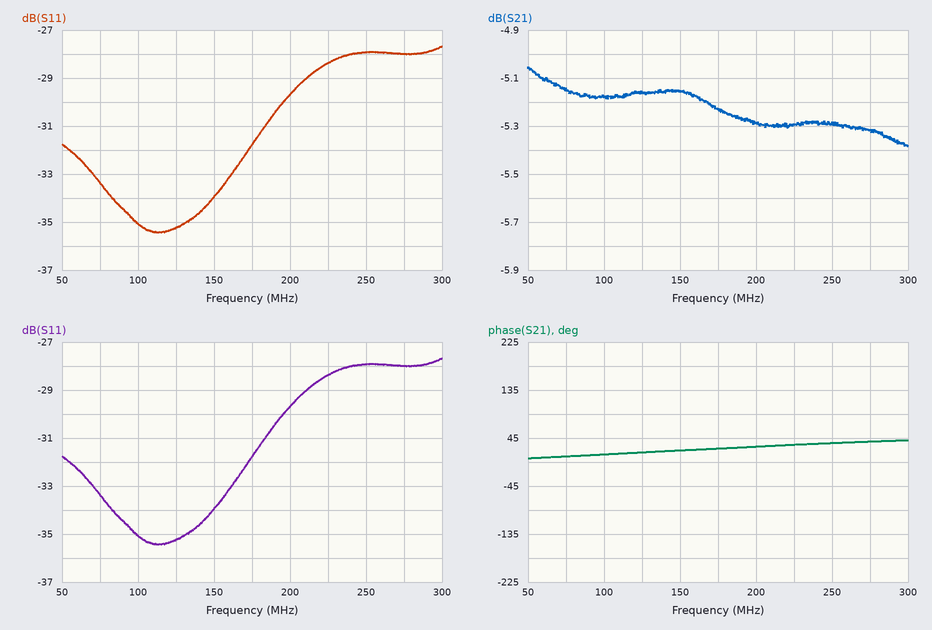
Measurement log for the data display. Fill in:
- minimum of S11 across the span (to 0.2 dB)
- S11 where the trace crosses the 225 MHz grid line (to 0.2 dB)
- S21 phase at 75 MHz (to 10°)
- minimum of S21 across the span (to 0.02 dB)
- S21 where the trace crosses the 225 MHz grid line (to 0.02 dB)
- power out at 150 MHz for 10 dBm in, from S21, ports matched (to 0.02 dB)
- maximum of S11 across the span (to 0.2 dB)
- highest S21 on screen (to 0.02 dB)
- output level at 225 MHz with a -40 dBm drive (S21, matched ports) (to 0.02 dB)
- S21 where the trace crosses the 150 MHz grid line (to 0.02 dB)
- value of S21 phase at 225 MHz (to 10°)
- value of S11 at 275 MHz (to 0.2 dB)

-35.4 dB
-28.4 dB
10°
-5.38 dB
-5.30 dB
4.84 dBm
-27.6 dB
-5.06 dB
-45.30 dBm
-5.16 dB
30°
-28.0 dB
